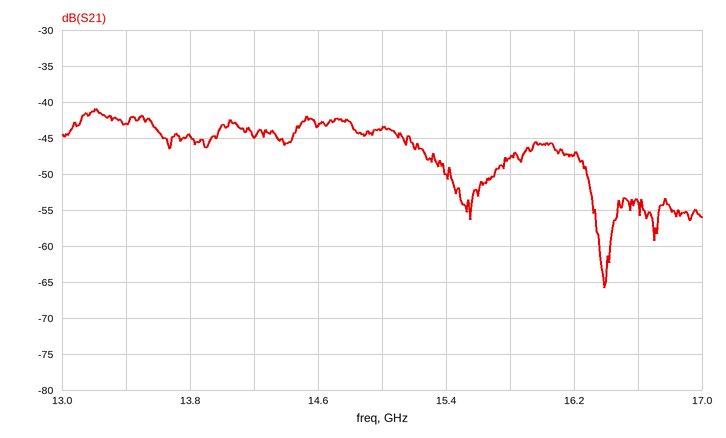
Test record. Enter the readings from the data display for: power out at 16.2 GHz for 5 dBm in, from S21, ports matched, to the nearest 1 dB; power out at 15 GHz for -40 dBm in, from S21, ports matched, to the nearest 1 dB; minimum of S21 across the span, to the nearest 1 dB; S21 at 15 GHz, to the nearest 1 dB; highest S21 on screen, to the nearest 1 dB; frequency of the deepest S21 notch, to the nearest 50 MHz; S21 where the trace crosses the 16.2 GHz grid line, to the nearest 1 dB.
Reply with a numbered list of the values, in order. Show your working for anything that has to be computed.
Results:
1. 5 dBm + (-47 dB) = -42 dBm
2. -40 dBm + (-44 dB) = -84 dBm
3. -66 dB
4. -44 dB
5. -41 dB
6. 16.40 GHz
7. -47 dB
